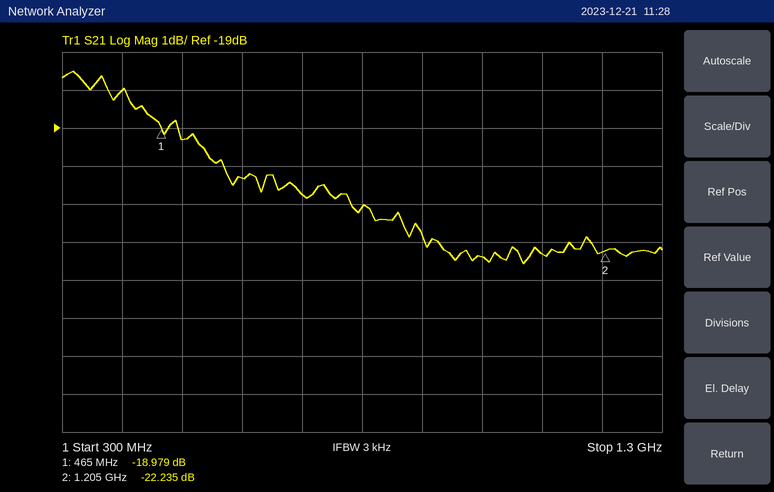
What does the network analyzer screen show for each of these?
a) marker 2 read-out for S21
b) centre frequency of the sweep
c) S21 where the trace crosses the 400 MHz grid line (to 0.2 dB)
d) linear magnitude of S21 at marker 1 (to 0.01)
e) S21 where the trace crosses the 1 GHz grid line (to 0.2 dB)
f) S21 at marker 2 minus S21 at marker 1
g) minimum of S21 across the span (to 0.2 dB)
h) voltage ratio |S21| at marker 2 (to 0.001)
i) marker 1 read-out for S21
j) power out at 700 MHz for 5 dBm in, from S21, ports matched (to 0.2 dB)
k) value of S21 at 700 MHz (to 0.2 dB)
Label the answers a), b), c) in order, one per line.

a) -22.235 dB
b) 800 MHz
c) -18.0 dB
d) 0.11
e) -22.4 dB
f) -3.256 dB
g) -22.6 dB
h) 0.077
i) -18.979 dB
j) -15.8 dBm
k) -20.8 dB
